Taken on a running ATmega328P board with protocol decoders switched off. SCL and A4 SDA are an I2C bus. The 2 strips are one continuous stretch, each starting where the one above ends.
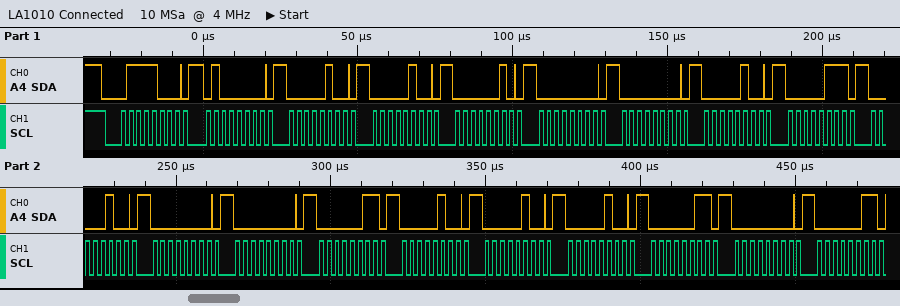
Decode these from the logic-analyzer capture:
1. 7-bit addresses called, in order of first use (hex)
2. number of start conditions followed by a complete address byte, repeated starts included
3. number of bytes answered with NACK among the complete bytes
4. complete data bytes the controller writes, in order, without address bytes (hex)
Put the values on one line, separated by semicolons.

0x3C; 1; 0; 40 04 04 02 00 00 04 07 04 00 00 03 04 04 04 03 00 03
